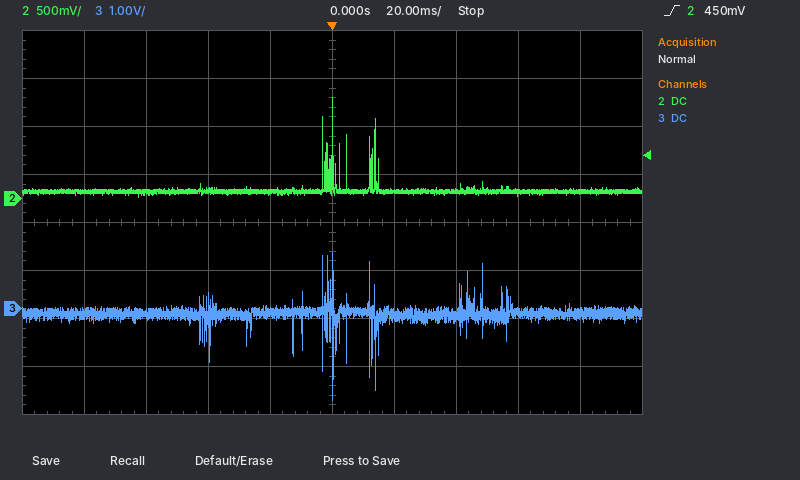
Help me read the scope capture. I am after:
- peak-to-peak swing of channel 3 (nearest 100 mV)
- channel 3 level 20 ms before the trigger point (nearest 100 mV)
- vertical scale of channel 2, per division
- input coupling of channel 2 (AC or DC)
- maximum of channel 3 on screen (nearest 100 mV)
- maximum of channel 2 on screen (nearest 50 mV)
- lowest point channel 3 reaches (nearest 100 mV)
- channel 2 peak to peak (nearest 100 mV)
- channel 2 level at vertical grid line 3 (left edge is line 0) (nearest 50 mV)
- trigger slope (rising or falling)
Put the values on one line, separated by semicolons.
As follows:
3.1 V; -100 mV; 500 mV; DC; 1.2 V; 1.05 V; -1.9 V; 1.00 V; 100 mV; rising
